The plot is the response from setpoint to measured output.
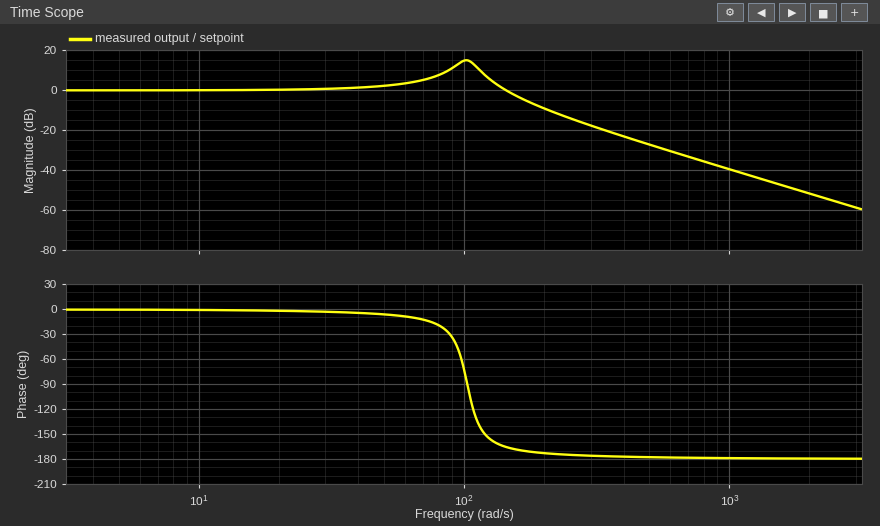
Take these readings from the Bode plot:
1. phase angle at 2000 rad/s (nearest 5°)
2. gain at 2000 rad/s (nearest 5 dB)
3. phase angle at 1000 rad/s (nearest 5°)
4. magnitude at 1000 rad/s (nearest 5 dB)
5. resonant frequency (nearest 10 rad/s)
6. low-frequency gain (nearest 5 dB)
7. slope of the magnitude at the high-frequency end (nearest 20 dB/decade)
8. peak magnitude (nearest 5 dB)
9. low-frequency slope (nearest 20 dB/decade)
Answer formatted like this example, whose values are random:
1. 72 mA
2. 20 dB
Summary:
1. -180°
2. -50 dB
3. -180°
4. -40 dB
5. 100 rad/s
6. 0 dB
7. -40 dB/decade
8. 15 dB
9. 0 dB/decade
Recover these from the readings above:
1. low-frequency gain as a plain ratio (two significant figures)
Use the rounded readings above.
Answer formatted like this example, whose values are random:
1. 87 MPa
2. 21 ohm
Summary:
1. 1.0
